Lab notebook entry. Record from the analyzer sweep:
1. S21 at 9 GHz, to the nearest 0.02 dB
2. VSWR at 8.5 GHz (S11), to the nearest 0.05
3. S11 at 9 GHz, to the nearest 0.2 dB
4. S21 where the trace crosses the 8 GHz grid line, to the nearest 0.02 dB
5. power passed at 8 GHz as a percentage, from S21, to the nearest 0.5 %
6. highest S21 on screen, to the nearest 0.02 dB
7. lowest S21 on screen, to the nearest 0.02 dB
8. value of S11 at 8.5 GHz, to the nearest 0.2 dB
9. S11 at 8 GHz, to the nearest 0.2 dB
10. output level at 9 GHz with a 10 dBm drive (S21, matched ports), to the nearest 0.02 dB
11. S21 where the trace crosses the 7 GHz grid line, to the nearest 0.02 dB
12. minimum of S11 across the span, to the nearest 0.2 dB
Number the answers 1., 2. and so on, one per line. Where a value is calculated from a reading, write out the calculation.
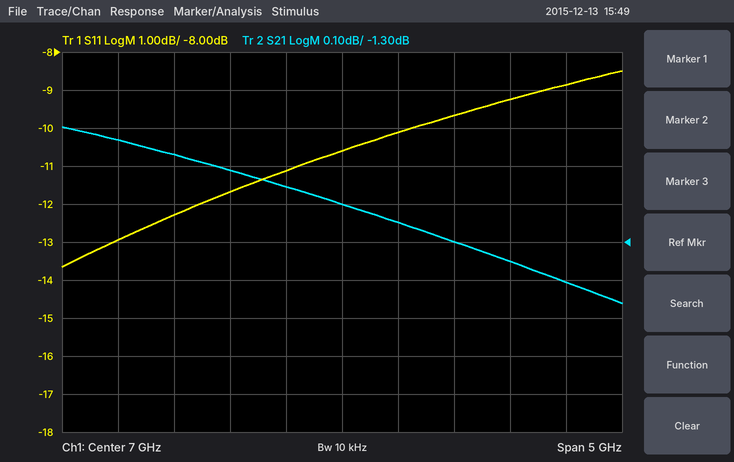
1. -1.40 dB
2. |Γ| = 10^(-9.2/20) = 0.3467; VSWR = (1 + 0.3467)/(1 − 0.3467) ≈ 2.06, so 2.05 to the nearest 0.05
3. -8.8 dB
4. -1.30 dB
5. 10^(-1.3/10) ≈ 74.1 %, so 74.0 % to the nearest 0.5 %
6. -1.00 dB
7. -1.46 dB
8. -9.2 dB
9. -9.6 dB
10. 10 dBm + (-1.40 dB) = 8.60 dBm
11. -1.20 dB
12. -13.6 dB
